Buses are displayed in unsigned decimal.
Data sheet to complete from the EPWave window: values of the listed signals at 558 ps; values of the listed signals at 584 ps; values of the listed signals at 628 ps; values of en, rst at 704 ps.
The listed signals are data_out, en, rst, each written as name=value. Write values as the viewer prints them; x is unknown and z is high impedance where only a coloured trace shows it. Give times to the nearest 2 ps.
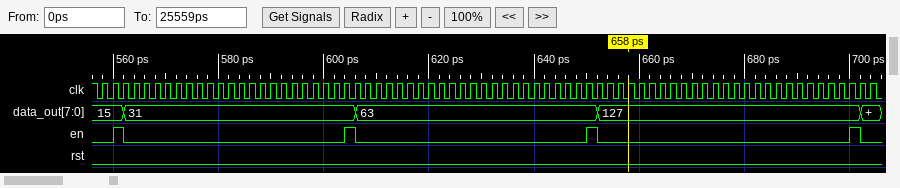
data_out=15, en=0, rst=0
data_out=31, en=0, rst=0
data_out=63, en=0, rst=0
en=0, rst=0
